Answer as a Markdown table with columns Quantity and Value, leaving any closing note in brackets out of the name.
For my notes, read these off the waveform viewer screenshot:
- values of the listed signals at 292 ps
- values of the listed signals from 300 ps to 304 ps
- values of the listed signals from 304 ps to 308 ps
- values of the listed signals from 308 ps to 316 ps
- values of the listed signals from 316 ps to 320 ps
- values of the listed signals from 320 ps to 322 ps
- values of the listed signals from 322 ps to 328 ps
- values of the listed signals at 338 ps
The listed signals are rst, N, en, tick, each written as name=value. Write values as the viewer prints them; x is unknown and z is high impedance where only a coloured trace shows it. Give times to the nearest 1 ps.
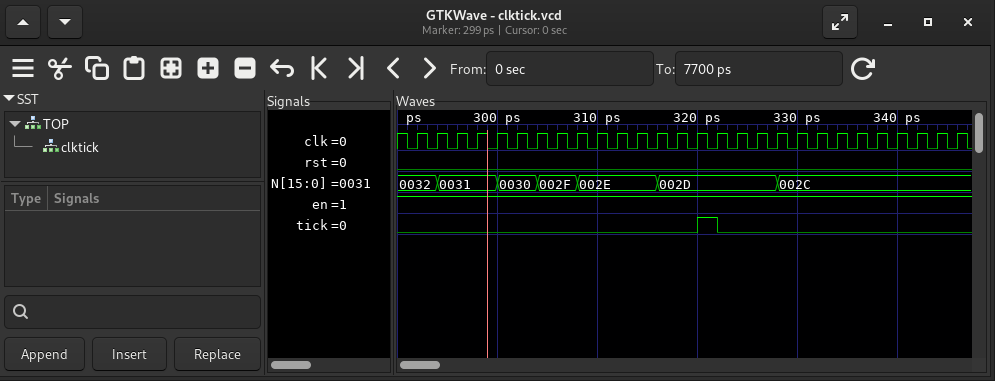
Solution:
| Quantity | Value |
|---|---|
| values of the listed signals at 292 ps | rst=0, N=0032, en=1, tick=0 |
| values of the listed signals from 300 ps to 304 ps | rst=0, N=0030, en=1, tick=0 |
| values of the listed signals from 304 ps to 308 ps | rst=0, N=002F, en=1, tick=0 |
| values of the listed signals from 308 ps to 316 ps | rst=0, N=002E, en=1, tick=0 |
| values of the listed signals from 316 ps to 320 ps | rst=0, N=002D, en=1, tick=0 |
| values of the listed signals from 320 ps to 322 ps | rst=0, N=002D, en=1, tick=1 |
| values of the listed signals from 322 ps to 328 ps | rst=0, N=002D, en=1, tick=0 |
| values of the listed signals at 338 ps | rst=0, N=002C, en=1, tick=0 |
